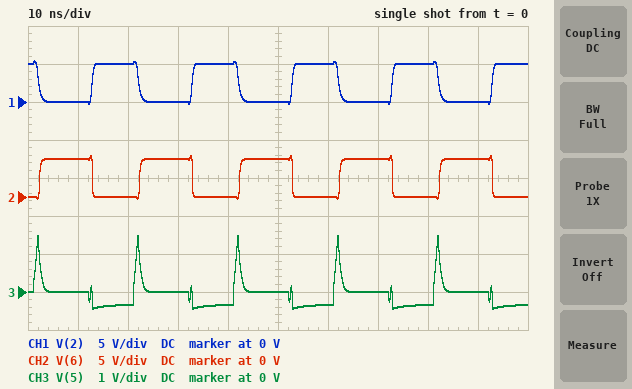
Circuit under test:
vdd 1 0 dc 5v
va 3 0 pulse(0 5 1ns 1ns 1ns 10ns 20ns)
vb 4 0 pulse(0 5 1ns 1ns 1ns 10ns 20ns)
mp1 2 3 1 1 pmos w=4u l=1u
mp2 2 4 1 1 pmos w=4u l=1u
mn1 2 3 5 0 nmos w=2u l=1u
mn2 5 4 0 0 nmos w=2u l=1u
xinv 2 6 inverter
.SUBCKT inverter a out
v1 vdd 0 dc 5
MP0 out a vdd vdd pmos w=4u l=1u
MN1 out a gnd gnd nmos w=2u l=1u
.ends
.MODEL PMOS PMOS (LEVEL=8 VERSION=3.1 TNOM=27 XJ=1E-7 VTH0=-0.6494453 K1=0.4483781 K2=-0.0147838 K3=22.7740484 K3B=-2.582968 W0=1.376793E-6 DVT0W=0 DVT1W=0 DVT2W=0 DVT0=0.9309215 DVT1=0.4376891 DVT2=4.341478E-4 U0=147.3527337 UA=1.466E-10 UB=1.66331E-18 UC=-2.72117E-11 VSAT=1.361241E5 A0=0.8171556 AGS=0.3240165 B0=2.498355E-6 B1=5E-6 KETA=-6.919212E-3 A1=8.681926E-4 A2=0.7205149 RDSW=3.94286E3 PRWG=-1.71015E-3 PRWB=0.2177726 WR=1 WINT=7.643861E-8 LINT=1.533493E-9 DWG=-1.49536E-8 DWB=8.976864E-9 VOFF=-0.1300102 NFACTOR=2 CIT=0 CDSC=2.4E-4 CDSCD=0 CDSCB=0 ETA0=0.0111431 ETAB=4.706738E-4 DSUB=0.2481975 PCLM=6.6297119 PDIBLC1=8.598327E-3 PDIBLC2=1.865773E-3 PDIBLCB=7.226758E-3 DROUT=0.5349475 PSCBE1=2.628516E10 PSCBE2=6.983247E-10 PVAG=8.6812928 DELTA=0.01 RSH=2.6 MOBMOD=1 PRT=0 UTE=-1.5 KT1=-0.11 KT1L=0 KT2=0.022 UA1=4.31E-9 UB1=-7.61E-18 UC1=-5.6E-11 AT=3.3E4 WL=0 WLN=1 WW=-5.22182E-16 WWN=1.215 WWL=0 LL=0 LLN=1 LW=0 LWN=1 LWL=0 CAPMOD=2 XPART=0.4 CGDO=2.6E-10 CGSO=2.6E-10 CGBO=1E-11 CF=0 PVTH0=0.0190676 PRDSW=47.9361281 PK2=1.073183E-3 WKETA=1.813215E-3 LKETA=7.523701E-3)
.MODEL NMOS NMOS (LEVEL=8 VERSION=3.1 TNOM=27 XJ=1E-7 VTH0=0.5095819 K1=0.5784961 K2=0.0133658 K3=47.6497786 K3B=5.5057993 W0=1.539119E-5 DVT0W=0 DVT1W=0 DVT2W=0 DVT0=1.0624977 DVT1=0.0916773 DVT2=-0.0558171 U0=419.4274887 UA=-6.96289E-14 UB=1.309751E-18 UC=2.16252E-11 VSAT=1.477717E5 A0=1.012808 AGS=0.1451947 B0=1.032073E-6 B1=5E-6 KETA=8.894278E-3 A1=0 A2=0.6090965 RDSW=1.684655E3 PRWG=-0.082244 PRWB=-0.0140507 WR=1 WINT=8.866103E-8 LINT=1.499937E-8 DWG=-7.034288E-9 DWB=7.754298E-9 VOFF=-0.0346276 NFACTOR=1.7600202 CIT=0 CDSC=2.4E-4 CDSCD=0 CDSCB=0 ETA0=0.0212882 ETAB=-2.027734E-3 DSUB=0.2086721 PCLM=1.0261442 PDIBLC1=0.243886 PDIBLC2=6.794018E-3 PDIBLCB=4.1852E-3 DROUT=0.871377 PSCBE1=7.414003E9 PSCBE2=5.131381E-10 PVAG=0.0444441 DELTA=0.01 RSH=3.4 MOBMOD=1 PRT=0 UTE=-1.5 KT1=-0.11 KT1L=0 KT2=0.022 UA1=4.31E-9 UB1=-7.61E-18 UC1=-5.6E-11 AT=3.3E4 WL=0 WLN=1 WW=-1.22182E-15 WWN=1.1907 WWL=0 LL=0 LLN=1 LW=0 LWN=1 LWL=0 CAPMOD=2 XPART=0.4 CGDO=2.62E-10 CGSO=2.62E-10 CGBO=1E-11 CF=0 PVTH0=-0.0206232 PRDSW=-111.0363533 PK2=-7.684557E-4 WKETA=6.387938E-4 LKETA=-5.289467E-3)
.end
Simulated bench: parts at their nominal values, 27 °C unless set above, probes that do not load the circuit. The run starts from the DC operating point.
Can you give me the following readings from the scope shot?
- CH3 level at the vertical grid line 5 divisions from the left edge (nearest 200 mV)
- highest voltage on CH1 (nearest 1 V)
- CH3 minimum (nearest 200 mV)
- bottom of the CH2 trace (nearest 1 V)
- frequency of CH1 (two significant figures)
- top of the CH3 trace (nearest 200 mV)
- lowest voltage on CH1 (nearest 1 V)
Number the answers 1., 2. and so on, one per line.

1. 0 V
2. 5 V
3. -400 mV
4. 0 V
5. 50 MHz
6. 1.4 V
7. 0 V
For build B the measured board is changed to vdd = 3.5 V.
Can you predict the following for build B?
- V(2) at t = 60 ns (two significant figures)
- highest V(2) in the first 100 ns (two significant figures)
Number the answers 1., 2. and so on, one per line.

1. 3.5 V
2. 3.8 V
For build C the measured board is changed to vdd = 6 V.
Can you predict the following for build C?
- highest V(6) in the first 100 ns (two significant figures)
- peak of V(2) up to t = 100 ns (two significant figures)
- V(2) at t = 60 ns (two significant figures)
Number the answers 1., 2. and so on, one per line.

1. 5.3 V
2. 6.3 V
3. 6.0 V
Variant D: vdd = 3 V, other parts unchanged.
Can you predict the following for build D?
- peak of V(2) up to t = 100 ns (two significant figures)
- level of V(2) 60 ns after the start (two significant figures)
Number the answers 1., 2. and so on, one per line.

1. 3.3 V
2. 3.0 V
